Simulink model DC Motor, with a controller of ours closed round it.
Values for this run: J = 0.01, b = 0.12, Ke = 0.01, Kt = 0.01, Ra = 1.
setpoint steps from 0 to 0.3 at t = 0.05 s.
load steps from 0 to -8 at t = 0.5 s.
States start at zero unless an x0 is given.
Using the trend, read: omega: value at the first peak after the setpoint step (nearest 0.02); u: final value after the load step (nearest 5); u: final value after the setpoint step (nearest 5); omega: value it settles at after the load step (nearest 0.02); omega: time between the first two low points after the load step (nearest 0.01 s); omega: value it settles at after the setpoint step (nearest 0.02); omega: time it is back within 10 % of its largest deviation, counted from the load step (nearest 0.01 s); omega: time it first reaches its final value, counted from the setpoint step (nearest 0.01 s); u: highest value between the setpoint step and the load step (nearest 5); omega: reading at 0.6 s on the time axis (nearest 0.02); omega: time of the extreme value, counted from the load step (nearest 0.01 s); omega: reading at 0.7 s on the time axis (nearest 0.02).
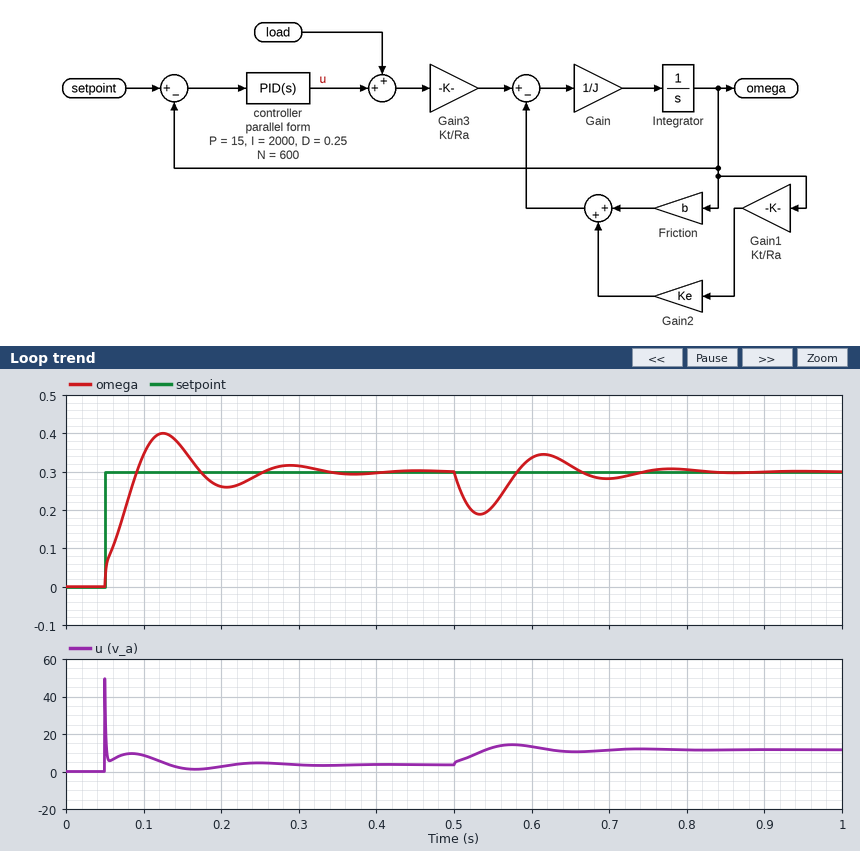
0.40
10
5
0.30
0.16 s
0.30
0.22 s
0.04 s
50
0.34
0.03 s
0.28
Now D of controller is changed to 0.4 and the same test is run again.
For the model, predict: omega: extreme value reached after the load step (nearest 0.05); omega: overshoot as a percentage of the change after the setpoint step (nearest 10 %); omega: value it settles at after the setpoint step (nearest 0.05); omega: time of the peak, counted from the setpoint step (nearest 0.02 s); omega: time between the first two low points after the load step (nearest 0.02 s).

0.20
30 %
0.30
0.08 s
0.18 s
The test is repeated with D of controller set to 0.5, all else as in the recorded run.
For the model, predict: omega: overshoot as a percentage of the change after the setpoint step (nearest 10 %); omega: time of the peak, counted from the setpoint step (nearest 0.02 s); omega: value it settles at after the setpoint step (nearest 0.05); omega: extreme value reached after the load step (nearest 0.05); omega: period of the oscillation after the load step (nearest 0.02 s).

30 %
0.08 s
0.30
0.20
0.18 s
